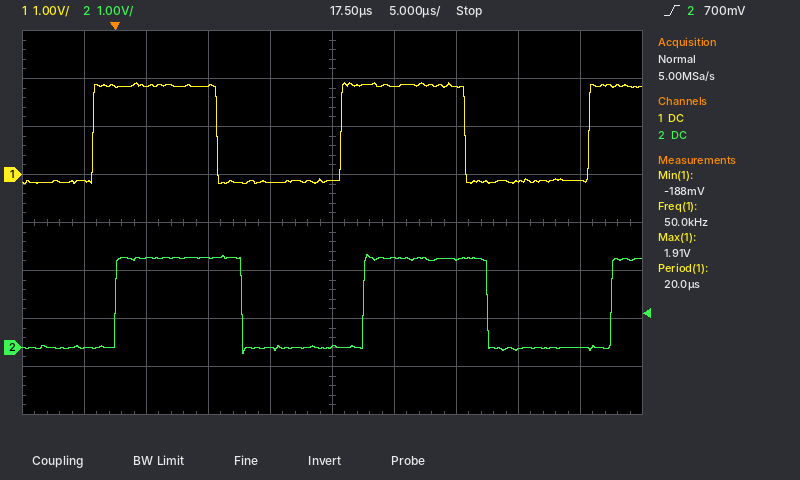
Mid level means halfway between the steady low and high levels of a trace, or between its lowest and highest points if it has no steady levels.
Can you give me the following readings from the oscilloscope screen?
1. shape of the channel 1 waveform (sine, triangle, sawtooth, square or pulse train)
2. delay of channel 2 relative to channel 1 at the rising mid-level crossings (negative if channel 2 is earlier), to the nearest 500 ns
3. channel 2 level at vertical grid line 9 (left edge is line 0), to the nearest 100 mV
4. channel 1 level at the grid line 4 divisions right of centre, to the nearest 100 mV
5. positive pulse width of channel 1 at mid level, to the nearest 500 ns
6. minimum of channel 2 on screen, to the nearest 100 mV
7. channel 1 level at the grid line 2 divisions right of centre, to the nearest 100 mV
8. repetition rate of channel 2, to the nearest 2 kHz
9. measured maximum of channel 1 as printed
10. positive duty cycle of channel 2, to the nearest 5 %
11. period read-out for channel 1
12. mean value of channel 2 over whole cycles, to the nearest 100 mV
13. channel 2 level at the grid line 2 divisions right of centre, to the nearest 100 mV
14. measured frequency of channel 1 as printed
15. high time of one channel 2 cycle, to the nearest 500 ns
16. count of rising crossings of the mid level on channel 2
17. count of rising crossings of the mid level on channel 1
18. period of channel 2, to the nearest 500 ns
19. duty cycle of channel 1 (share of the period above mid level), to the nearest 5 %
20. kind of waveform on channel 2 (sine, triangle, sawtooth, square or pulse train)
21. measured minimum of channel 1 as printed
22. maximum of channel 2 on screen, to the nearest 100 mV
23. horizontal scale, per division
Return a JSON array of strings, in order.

["square", "+2.0 µs", "0.0 V", "-100 mV", "10.0 µs", "-100 mV", "1.8 V", "50 kHz", "1.91 V", "50 %", "20.0 µs", "900 mV", "1.8 V", "50.0 kHz", "10.0 µs", "3", "3", "20.0 µs", "50 %", "square", "-188 mV", "1.9 V", "5 µs"]
